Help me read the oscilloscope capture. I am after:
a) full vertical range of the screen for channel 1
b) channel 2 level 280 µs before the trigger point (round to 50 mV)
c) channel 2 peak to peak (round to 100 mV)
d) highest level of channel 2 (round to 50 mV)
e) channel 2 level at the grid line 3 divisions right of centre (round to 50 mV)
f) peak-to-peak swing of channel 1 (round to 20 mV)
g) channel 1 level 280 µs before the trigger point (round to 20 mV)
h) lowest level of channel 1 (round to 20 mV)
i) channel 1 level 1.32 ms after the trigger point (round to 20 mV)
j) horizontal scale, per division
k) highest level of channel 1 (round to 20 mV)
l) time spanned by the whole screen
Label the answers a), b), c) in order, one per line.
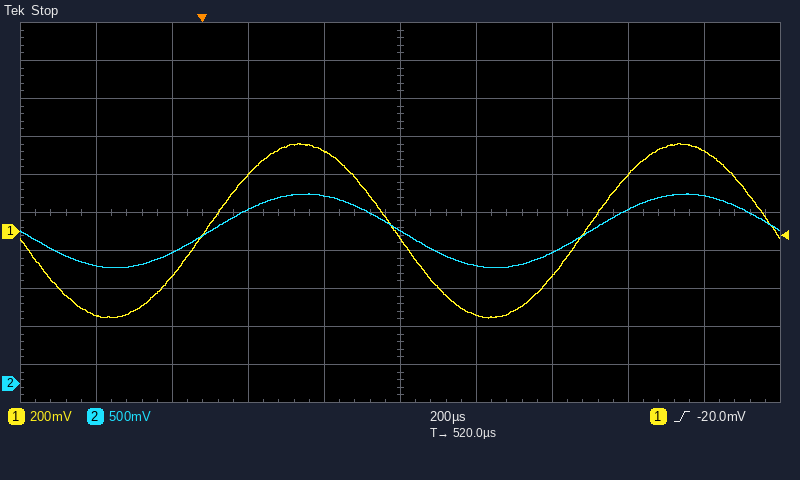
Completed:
a) 2 V
b) 1.55 V
c) 1.00 V
d) 2.50 V
e) 2.30 V
f) 920 mV
g) -440 mV
h) -460 mV
i) 420 mV
j) 200 µs
k) 460 mV
l) 2 ms
